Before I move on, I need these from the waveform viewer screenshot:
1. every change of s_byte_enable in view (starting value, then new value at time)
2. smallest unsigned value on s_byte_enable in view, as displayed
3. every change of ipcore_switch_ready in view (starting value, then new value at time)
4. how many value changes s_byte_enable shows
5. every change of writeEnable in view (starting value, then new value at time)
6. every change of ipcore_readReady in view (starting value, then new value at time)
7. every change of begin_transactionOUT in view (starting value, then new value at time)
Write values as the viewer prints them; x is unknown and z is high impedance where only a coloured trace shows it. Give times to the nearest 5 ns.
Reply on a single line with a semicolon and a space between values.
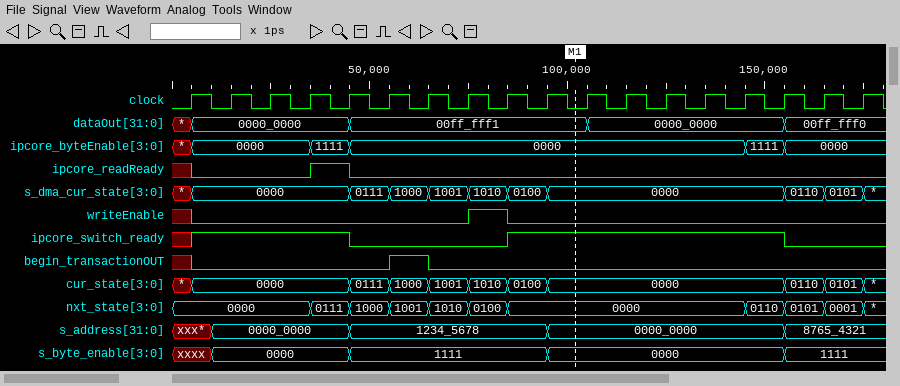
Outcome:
xxxx, 0000 at 10 ns, 1111 at 45 ns, 0000 at 95 ns, 1111 at 155 ns; 0000; x, 1 at 5 ns, 0 at 45 ns, 1 at 85 ns, 0 at 155 ns; 4; x, 0 at 5 ns, 1 at 75 ns, 0 at 85 ns; x, 0 at 5 ns, 1 at 35 ns, 0 at 45 ns; x, 0 at 5 ns, 1 at 55 ns, 0 at 65 ns
